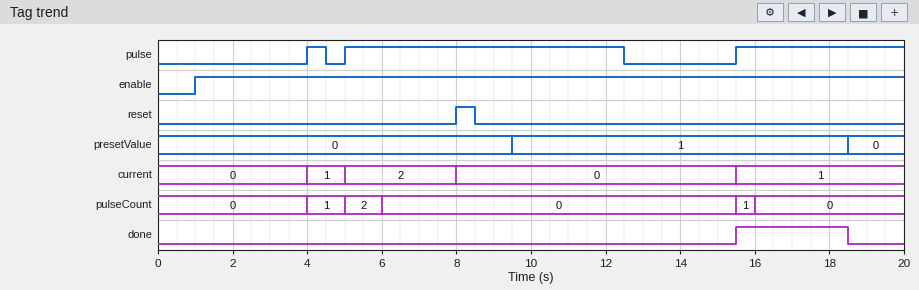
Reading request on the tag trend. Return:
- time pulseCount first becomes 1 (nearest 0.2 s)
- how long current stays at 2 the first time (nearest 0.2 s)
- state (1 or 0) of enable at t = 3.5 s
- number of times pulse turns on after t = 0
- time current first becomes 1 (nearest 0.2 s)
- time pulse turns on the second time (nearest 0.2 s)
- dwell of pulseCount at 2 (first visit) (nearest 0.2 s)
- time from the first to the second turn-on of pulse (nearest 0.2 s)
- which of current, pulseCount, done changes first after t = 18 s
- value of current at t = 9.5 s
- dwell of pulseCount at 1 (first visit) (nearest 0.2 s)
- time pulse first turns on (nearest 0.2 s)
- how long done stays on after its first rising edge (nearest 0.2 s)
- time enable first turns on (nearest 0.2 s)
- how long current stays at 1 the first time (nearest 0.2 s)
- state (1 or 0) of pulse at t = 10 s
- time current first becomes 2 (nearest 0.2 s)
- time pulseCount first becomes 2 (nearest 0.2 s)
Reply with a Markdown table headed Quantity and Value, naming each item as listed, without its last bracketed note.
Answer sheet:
| Quantity | Value |
|---|---|
| time pulseCount first becomes 1 | 4.0 s |
| how long current stays at 2 the first time | 3.0 s |
| state (1 or 0) of enable at t = 3.5 s | 1 |
| number of times pulse turns on after t = 0 | 3 |
| time current first becomes 1 | 4.0 s |
| time pulse turns on the second time | 5.0 s |
| dwell of pulseCount at 2 (first visit) | 1.0 s |
| time from the first to the second turn-on of pulse | 1.0 s |
| which of current, pulseCount, done changes first after t = 18 s | done |
| value of current at t = 9.5 s | 0 |
| dwell of pulseCount at 1 (first visit) | 1.0 s |
| time pulse first turns on | 4.0 s |
| how long done stays on after its first rising edge | 3.0 s |
| time enable first turns on | 1.0 s |
| how long current stays at 1 the first time | 1.0 s |
| state (1 or 0) of pulse at t = 10 s | 1 |
| time current first becomes 2 | 5.0 s |
| time pulseCount first becomes 2 | 5.0 s |
